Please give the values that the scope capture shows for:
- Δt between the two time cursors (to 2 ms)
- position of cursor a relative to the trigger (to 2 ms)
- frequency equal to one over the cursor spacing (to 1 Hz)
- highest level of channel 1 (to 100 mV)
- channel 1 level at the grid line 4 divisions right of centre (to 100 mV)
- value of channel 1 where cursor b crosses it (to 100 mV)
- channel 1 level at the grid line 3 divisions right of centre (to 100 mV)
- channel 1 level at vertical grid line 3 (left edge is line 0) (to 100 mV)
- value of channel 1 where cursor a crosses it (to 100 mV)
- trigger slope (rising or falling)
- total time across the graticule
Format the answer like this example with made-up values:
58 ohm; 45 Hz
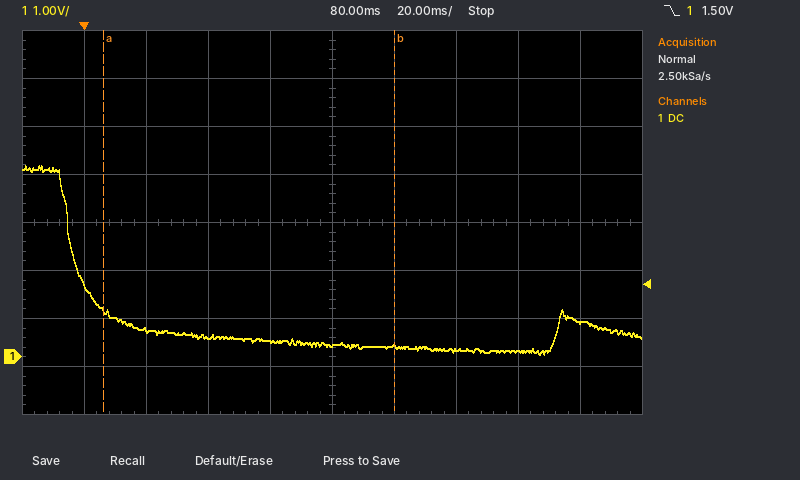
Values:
94 ms; +6 ms; 11 Hz; 4.0 V; 700 mV; 200 mV; 100 mV; 400 mV; 1.0 V; falling; 200 ms
